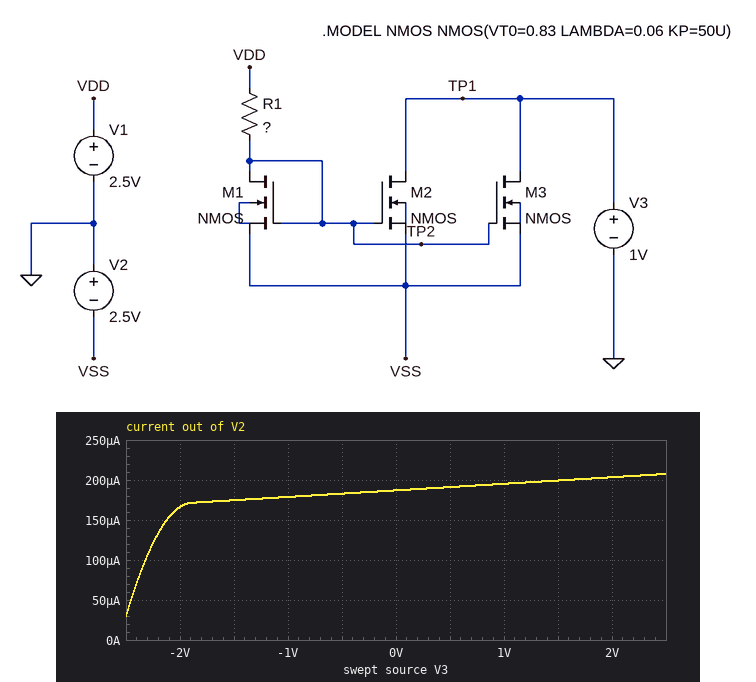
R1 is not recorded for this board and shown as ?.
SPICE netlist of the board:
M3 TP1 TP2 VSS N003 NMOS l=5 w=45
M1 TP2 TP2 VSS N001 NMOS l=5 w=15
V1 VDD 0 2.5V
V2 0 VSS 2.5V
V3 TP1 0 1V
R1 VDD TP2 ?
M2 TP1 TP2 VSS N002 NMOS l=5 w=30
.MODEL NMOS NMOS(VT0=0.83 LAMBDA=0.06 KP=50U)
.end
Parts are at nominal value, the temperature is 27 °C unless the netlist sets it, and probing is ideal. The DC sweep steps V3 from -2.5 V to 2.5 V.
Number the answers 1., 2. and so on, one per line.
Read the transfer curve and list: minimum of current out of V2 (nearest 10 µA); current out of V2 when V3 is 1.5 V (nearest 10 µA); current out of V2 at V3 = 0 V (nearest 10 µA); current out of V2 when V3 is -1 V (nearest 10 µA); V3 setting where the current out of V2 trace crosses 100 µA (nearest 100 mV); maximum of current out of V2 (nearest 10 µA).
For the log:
1. 30 µA
2. 200 µA
3. 190 µA
4. 180 µA
5. -2.3 V
6. 210 µA
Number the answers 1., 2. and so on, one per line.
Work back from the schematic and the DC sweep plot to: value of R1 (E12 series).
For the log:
1. 120 kΩ
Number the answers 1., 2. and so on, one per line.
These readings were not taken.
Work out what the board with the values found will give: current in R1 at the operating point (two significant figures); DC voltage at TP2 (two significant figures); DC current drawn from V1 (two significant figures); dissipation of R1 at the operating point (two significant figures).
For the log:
1. 30 µA
2. -1.1 V
3. 30 µA
4. 110 µW
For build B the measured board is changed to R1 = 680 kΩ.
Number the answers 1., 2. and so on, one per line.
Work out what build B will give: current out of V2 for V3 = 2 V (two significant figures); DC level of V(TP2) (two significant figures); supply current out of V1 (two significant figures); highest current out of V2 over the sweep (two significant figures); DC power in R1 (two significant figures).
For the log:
1. 40 µA
2. -1.4 V
3. 5.7 µA
4. 41 µA
5. 22 µW
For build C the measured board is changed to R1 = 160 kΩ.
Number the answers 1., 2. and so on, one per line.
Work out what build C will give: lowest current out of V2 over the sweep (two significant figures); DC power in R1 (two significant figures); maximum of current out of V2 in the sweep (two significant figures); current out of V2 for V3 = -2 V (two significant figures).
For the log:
1. 23 µA
2. 83 µW
3. 160 µA
4. 130 µA
